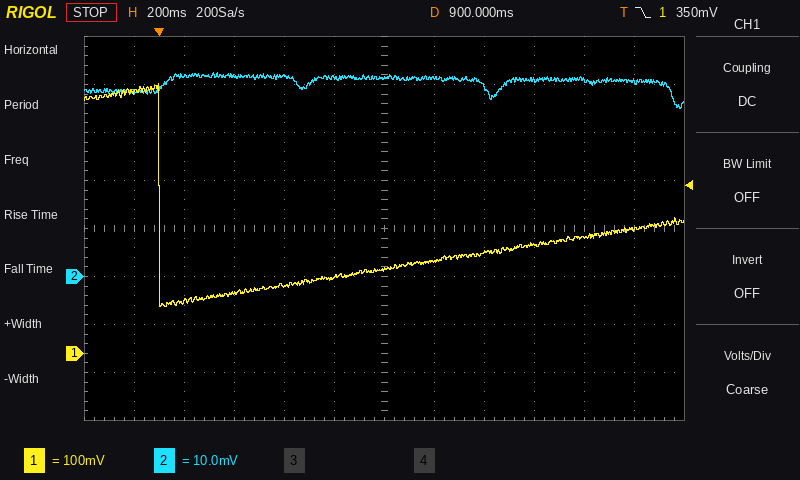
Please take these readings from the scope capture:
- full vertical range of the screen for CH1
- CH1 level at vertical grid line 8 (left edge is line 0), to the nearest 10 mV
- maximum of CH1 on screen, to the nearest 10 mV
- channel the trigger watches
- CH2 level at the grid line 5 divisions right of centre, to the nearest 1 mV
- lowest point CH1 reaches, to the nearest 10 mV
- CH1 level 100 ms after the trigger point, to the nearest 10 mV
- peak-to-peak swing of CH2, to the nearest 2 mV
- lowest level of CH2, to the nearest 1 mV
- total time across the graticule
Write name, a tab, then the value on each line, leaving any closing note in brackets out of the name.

full vertical range of the screen for CH1	800 mV
CH1 level at vertical grid line 8 (left edge is line 0), to the nearest 10 mV	210 mV
maximum of CH1 on screen, to the nearest 10 mV	560 mV
channel the trigger watches	CH1
CH2 level at the grid line 5 divisions right of centre, to the nearest 1 mV	41 mV
lowest point CH1 reaches, to the nearest 10 mV	100 mV
CH1 level 100 ms after the trigger point, to the nearest 10 mV	110 mV
peak-to-peak swing of CH2, to the nearest 2 mV	8 mV
lowest level of CH2, to the nearest 1 mV	35 mV
total time across the graticule	2.4 s
